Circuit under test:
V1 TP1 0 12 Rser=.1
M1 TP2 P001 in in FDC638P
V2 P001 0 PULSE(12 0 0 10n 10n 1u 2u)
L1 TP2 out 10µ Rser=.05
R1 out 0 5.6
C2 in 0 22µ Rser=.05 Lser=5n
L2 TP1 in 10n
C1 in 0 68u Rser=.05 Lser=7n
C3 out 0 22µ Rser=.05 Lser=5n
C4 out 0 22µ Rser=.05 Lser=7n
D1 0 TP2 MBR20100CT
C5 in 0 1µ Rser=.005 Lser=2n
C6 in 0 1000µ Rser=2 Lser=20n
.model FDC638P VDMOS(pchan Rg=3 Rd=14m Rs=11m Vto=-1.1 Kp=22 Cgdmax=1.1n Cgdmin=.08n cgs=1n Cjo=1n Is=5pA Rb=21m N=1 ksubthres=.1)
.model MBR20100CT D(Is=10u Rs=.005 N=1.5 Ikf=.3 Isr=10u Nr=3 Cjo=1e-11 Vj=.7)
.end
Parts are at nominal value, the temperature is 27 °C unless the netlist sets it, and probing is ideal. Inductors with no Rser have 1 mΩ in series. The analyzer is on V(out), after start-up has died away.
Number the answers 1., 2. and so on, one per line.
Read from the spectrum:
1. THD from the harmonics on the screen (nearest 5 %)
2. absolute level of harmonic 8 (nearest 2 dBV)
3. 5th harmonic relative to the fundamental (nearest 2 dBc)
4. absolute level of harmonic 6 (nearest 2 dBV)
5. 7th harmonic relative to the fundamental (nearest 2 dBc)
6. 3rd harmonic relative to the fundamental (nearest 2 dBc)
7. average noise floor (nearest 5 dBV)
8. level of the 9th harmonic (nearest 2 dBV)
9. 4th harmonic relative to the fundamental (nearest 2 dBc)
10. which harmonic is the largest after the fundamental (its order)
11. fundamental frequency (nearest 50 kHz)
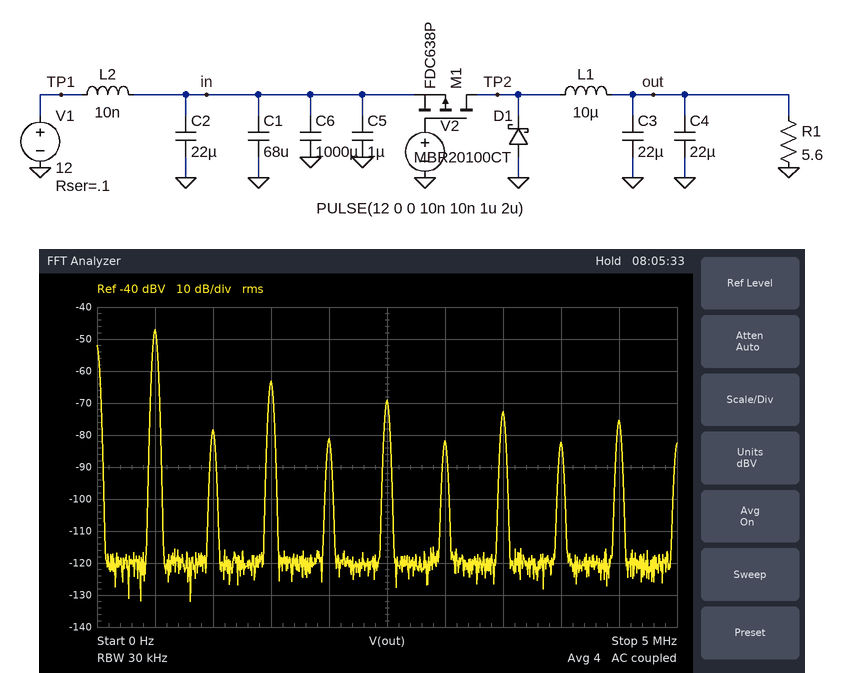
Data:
1. 20 %
2. -82 dBV
3. -22 dBc
4. -82 dBV
5. -26 dBc
6. -16 dBc
7. -120 dBV
8. -76 dBV
9. -34 dBc
10. 3
11. 500 kHz
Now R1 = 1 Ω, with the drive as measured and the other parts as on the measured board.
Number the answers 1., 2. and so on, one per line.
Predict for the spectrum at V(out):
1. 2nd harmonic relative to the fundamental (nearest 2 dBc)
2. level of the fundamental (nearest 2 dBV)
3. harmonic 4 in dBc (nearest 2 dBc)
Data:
1. -34 dBc
2. -48 dBV
3. -36 dBc
